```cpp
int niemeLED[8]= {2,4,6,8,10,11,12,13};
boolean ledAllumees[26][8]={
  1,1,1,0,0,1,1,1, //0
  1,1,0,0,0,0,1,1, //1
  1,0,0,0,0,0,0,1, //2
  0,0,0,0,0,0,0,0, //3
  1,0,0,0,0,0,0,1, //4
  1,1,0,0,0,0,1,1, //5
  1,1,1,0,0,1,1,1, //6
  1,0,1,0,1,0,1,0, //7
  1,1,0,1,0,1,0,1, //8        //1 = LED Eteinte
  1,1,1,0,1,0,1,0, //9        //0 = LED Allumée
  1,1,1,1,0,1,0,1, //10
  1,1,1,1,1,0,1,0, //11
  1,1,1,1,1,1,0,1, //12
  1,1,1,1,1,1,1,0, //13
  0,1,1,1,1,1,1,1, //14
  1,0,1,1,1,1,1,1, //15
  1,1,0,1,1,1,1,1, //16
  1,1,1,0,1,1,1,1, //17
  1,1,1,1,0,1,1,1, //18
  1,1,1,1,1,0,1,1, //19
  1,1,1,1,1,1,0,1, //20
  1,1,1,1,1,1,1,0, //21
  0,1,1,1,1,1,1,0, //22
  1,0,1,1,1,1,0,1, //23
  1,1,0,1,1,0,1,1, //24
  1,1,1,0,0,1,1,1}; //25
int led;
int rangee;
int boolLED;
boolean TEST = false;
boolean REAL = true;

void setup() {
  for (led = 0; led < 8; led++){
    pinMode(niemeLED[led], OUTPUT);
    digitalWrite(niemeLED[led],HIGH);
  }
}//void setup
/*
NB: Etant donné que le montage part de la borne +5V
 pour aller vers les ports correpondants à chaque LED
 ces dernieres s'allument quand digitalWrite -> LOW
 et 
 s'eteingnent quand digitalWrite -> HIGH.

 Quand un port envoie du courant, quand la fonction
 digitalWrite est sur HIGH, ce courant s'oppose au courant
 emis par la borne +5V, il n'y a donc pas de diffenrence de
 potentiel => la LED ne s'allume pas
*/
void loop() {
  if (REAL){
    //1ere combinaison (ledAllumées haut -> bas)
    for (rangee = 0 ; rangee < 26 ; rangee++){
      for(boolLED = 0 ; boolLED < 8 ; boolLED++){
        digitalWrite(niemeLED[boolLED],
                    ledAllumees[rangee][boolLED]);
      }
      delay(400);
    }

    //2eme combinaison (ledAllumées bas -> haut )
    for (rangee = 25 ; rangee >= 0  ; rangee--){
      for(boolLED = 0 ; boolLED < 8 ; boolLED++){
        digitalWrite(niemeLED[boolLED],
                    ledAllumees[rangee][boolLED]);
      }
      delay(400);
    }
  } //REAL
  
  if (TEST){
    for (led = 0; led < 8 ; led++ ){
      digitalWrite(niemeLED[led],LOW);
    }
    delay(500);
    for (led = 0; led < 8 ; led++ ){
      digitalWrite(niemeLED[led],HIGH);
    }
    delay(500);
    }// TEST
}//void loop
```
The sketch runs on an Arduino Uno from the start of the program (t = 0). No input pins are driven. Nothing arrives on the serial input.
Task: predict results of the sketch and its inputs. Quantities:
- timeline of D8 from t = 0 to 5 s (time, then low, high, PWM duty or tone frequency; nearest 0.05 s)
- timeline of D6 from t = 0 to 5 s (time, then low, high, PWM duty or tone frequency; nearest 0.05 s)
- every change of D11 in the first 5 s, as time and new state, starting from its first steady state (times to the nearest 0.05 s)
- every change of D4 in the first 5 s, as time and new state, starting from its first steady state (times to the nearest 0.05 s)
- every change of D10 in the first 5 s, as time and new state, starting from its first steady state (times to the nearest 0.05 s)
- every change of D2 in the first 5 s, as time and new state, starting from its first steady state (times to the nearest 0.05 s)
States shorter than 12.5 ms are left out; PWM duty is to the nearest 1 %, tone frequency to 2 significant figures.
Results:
0 s low; 3.2 s high; 3.6 s low; 4 s high
0 s high; 0.4 s low; 2.4 s high; 3.2 s low; 3.6 s high
0 s high; 0.4 s low; 2.4 s high; 2.8 s low; 3.2 s high; 3.6 s low; 4 s high; 4.4 s low; 4.8 s high
0 s high; 0.8 s low; 2 s high; 2.8 s low; 3.2 s high
0 s low; 2.8 s high; 3.2 s low; 3.6 s high; 4 s low; 4.4 s high
0 s high; 1.2 s low; 1.6 s high
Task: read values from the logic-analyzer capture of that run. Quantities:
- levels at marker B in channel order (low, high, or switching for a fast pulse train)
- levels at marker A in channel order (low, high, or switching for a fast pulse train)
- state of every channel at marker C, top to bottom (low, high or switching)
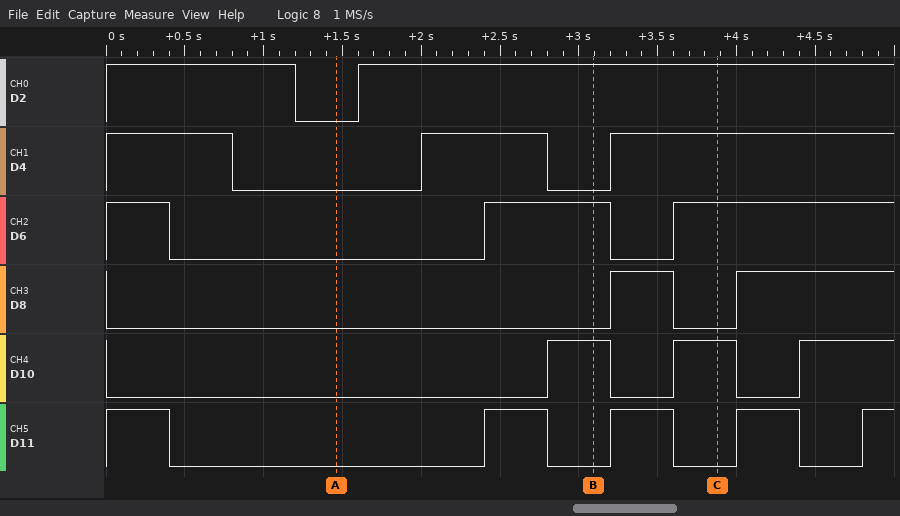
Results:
D2 high, D4 low, D6 high, D8 low, D10 high, D11 low
D2 low, D4 low, D6 low, D8 low, D10 low, D11 low
D2 high, D4 high, D6 high, D8 low, D10 high, D11 low
